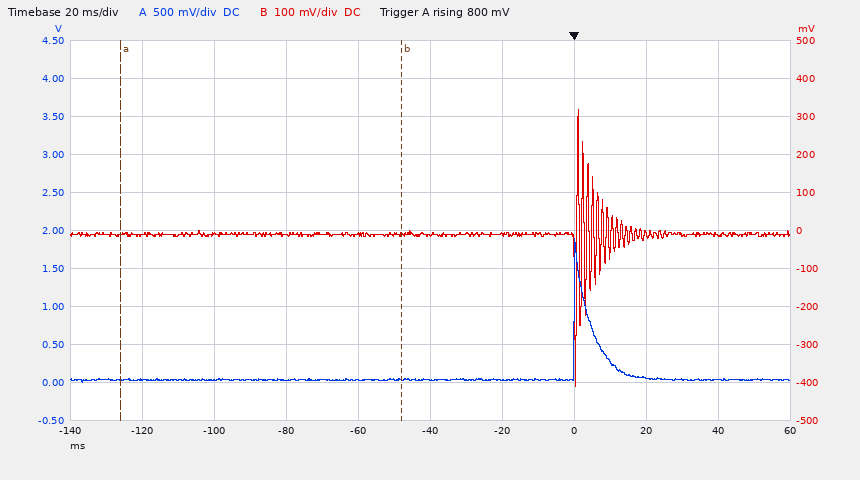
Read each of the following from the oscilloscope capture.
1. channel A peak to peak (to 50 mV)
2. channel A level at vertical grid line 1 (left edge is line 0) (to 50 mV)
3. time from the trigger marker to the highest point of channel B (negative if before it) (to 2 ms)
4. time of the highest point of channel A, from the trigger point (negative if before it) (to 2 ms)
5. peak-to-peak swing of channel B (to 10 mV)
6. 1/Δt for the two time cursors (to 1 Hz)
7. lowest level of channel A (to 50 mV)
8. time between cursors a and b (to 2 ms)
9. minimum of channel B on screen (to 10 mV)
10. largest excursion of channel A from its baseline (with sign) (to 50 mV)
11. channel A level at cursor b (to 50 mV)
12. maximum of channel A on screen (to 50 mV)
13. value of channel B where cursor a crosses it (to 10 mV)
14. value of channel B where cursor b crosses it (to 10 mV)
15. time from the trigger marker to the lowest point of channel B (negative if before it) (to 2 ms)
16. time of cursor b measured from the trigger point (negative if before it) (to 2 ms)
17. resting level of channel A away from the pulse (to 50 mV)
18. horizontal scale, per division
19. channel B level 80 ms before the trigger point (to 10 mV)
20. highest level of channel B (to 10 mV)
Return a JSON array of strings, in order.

["1.90 V", "50 mV", "+2 ms", "0 ms", "730 mV", "13 Hz", "0 mV", "78 ms", "-410 mV", "+1.85 V", "50 mV", "1.90 V", "-10 mV", "-10 mV", "0 ms", "-48 ms", "50 mV", "20 ms", "-10 mV", "320 mV"]
